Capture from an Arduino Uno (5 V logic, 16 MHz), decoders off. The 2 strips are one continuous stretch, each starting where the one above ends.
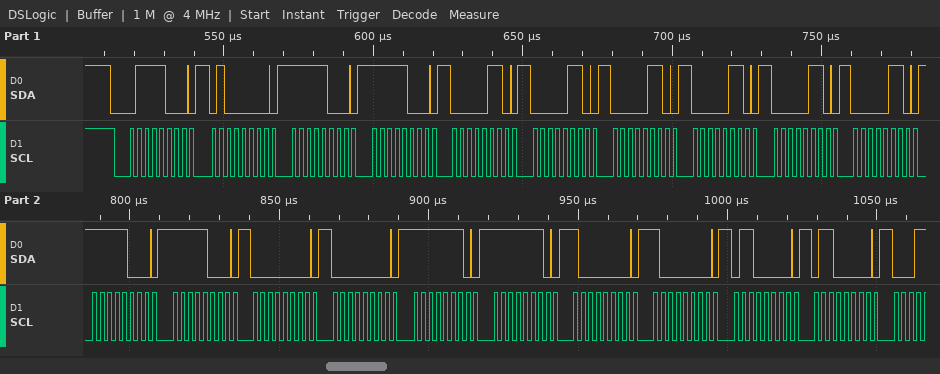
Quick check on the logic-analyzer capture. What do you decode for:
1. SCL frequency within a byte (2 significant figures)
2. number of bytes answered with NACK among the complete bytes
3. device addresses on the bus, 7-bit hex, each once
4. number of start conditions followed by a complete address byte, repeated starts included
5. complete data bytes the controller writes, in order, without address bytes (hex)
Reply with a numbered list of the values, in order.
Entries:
1. 400 kHz
2. 0
3. 0x3C
4. 1
5. 40 F8 F8 06 06 06 06 06 06 F8 F8 00 00 FE FE 80 80 60 60
